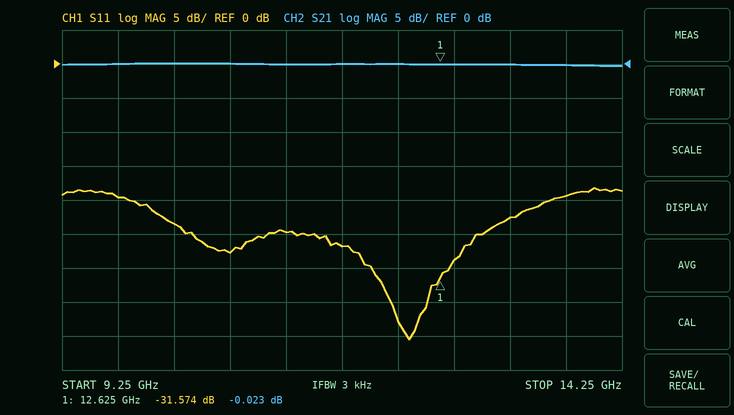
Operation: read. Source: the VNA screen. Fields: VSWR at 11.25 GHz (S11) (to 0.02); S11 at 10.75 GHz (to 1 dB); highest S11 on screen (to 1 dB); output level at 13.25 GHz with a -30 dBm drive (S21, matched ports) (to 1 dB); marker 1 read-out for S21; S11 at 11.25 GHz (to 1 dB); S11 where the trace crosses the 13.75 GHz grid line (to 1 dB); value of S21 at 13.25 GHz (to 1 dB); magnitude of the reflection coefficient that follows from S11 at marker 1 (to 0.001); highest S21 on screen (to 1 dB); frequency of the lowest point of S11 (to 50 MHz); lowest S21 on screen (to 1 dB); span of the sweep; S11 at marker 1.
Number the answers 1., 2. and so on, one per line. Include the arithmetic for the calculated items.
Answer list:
1. |Γ| = 10^(-25/20) = 0.0562; VSWR = (1 + 0.0562)/(1 − 0.0562) ≈ 1.12
2. -28 dB
3. -18 dB
4. -30 dBm + (0 dB) = -30 dBm
5. -0.023 dB
6. -25 dB
7. -19 dB
8. 0 dB
9. 10^(-31.574/20) ≈ 0.026
10. 0 dB
11. 12.35 GHz
12. 0 dB
13. 5 GHz
14. -31.574 dB
